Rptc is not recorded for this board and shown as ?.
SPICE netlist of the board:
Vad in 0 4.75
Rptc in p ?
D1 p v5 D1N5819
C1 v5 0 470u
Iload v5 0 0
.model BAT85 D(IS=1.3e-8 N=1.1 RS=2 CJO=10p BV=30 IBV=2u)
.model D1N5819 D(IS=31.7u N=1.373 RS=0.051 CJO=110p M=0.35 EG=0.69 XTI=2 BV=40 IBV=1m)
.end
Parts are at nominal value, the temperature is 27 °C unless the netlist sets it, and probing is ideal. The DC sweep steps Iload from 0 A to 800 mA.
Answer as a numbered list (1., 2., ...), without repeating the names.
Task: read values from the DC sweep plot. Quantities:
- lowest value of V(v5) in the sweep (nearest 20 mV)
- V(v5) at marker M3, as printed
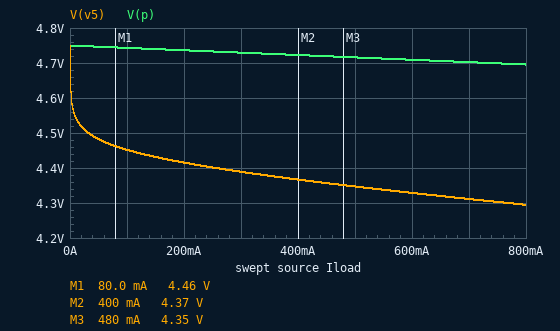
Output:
1. 4.30 V
2. 4.35 V
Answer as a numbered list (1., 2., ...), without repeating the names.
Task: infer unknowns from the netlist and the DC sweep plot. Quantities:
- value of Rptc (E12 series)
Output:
1. 0.068 Ω
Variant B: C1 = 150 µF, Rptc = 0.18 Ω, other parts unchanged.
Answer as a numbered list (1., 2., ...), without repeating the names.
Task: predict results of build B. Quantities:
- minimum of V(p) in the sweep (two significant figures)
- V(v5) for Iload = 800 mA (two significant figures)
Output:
1. 4.6 V
2. 4.2 V
